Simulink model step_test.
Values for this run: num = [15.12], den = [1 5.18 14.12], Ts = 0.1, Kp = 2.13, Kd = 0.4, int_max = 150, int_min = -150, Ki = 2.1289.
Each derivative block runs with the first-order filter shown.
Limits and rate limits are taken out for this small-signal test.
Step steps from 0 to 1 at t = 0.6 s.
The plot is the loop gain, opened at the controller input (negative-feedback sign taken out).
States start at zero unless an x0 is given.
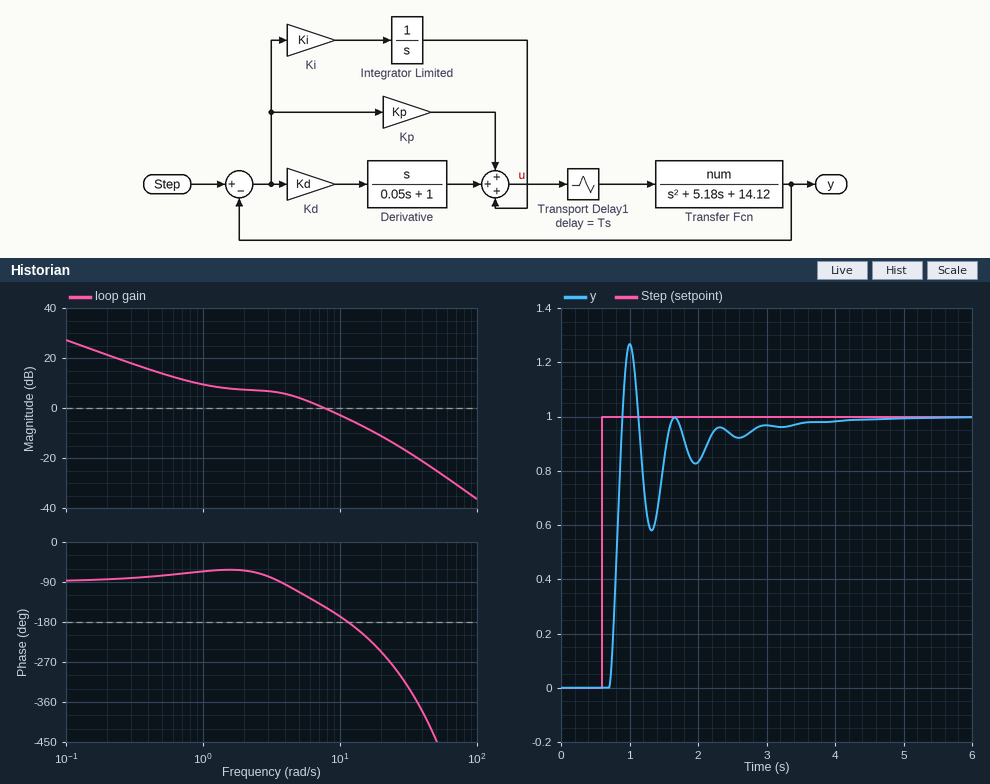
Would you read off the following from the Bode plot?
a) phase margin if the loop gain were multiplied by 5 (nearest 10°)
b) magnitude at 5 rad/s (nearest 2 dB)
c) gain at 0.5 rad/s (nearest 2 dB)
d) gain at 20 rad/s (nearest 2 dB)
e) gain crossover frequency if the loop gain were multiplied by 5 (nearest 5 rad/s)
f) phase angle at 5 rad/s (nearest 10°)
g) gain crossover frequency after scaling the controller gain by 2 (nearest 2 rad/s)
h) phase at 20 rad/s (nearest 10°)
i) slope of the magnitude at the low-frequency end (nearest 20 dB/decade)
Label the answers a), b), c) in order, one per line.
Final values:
a) -100°
b) 4 dB
c) 14 dB
d) -12 dB
e) 25 rad/s
f) -110°
g) 14 rad/s
h) -250°
i) -20 dB/decade
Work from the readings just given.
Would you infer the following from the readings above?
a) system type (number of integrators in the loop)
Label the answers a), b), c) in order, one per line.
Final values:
a) 1
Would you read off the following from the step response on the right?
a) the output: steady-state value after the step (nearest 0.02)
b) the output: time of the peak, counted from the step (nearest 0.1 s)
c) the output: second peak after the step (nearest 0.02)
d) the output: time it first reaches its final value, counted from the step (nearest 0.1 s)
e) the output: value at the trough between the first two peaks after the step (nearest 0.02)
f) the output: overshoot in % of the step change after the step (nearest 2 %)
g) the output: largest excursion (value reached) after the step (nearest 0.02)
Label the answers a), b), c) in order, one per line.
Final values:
a) 1.00
b) 0.4 s
c) 1.00
d) 0.3 s
e) 0.58
f) 26 %
g) 1.26
